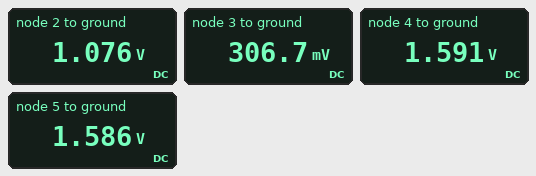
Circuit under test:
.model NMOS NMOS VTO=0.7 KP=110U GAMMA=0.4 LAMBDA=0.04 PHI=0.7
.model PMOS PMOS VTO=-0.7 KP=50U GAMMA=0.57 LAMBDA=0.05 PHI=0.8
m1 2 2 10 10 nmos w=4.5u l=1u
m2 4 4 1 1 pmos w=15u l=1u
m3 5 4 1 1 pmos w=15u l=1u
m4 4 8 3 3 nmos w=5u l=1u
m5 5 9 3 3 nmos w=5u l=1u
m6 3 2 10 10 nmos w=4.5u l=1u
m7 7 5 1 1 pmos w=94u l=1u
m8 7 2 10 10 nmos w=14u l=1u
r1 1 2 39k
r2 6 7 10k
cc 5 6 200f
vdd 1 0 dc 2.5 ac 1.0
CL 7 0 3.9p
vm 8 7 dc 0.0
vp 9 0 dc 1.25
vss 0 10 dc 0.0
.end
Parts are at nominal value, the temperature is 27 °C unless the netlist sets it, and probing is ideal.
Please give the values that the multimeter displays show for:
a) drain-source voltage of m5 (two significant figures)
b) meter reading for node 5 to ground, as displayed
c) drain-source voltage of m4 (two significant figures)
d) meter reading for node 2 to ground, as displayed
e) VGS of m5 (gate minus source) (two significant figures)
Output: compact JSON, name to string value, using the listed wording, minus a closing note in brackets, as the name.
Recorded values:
{"drain-source voltage of m5": "1.3 V", "meter reading for node 5 to ground, as displayed": "1.586 V", "drain-source voltage of m4": "1.3 V", "meter reading for node 2 to ground, as displayed": "1.076 V", "VGS of m5 (gate minus source)": "940 mV"}
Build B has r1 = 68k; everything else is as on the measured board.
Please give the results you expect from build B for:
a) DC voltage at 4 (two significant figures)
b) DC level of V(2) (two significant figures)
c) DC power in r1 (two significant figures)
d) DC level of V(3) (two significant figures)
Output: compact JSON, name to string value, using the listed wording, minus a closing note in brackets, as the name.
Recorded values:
{"DC voltage at 4": "1.6 V", "DC level of V(2)": "990 mV", "DC power in r1": "33 µW", "DC level of V(3)": "360 mV"}
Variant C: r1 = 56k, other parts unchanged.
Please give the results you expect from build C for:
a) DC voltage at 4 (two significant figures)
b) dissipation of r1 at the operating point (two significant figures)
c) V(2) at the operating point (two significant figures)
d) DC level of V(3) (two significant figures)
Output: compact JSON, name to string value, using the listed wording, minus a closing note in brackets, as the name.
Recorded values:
{"DC voltage at 4": "1.6 V", "dissipation of r1 at the operating point": "39 µW", "V(2) at the operating point": "1.0 V", "DC level of V(3)": "340 mV"}
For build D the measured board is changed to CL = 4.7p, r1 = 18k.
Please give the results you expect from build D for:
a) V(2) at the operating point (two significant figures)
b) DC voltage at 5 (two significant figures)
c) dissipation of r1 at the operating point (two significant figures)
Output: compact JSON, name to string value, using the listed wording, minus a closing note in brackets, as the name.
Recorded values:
{"V(2) at the operating point": "1.2 V", "DC voltage at 5": "1.5 V", "dissipation of r1 at the operating point": "91 µW"}
